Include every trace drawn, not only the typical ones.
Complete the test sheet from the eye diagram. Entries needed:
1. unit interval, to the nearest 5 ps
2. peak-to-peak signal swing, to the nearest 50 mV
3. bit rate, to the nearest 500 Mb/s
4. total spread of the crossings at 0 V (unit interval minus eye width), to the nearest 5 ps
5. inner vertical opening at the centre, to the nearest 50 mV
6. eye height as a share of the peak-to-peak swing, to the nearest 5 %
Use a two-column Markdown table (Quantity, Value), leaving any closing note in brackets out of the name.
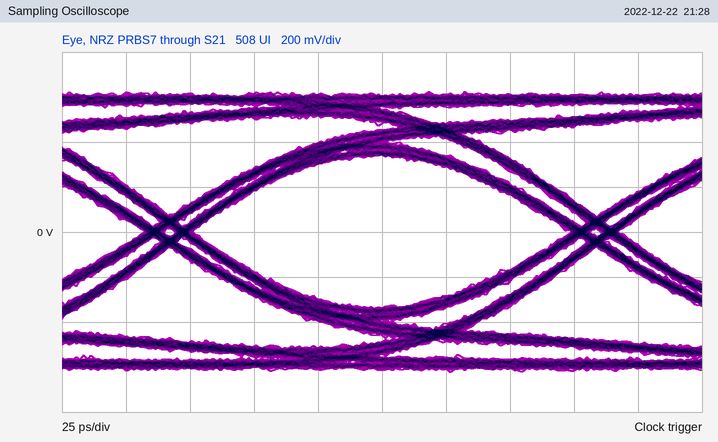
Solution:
| Quantity | Value |
|---|---|
| unit interval, to the nearest 5 ps | 165 ps |
| peak-to-peak signal swing, to the nearest 50 mV | 1.25 V |
| bit rate, to the nearest 500 Mb/s | 6.0 Gb/s |
| total spread of the crossings at 0 V (unit interval minus eye width), to the nearest 5 ps | 20 ps |
| inner vertical opening at the centre, to the nearest 50 mV | 700 mV |
| eye height as a share of the peak-to-peak swing, to the nearest 5 % | 55 % |
